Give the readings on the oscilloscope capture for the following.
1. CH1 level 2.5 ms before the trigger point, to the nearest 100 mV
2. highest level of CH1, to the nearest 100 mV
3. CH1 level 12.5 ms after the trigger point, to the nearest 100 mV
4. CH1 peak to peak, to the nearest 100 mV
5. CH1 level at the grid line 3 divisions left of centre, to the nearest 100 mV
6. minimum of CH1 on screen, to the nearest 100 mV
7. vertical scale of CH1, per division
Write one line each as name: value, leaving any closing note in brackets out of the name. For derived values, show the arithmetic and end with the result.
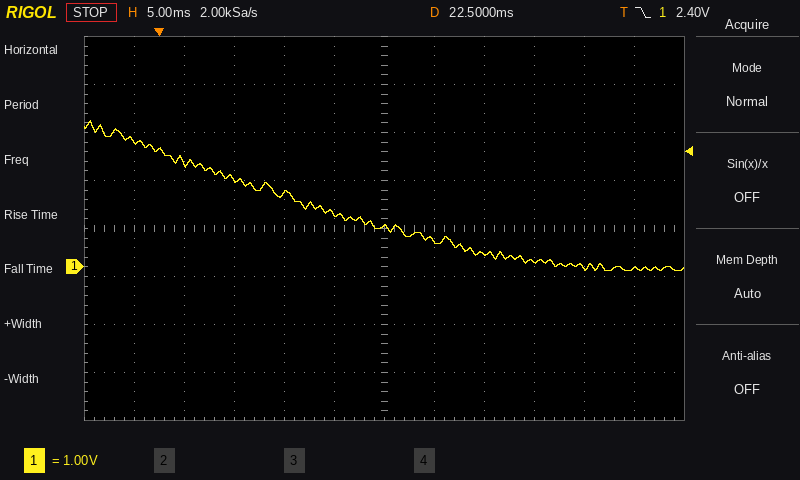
CH1 level 2.5 ms before the trigger point, to the nearest 100 mV: 2.6 V
highest level of CH1, to the nearest 100 mV: 3.0 V
CH1 level 12.5 ms after the trigger point, to the nearest 100 mV: 1.5 V
CH1 peak to peak, to the nearest 100 mV: 3.0 V − (-100 mV) = 3.1 V
CH1 level at the grid line 3 divisions left of centre, to the nearest 100 mV: 1.8 V
minimum of CH1 on screen, to the nearest 100 mV: -100 mV
vertical scale of CH1, per division: 1 V
